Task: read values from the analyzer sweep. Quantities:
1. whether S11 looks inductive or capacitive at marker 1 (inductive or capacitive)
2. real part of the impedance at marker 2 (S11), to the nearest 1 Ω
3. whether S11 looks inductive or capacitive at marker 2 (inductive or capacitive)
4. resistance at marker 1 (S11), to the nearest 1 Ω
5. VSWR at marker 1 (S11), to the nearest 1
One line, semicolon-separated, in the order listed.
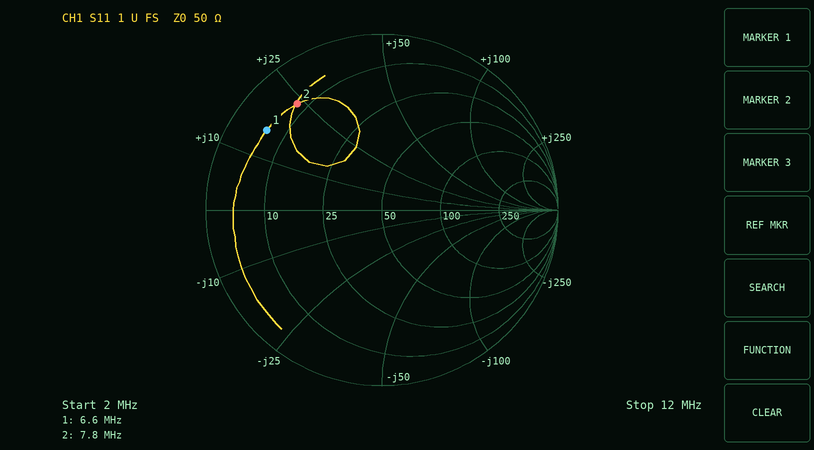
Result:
inductive; 8 Ω; inductive; 6 Ω; 9
